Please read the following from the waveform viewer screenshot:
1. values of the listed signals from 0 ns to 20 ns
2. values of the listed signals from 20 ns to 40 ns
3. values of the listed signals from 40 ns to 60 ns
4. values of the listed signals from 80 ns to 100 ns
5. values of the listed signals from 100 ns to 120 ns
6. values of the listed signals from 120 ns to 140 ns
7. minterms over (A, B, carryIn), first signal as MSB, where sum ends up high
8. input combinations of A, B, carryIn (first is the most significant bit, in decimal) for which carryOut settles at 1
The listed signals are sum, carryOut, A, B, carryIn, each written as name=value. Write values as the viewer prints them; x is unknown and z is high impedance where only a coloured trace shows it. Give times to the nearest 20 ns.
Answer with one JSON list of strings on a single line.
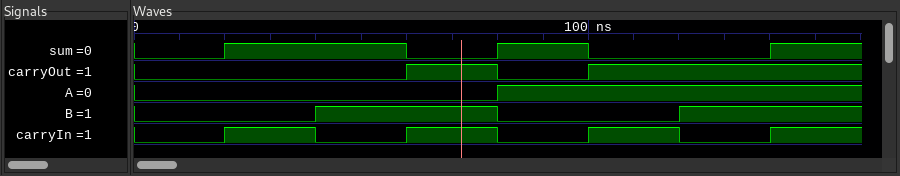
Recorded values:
["sum=0, carryOut=0, A=0, B=0, carryIn=0", "sum=1, carryOut=0, A=0, B=0, carryIn=1", "sum=1, carryOut=0, A=0, B=1, carryIn=0", "sum=1, carryOut=0, A=1, B=0, carryIn=0", "sum=0, carryOut=1, A=1, B=0, carryIn=1", "sum=0, carryOut=1, A=1, B=1, carryIn=0", "1, 2, 4, 7", "3, 5, 6, 7"]
